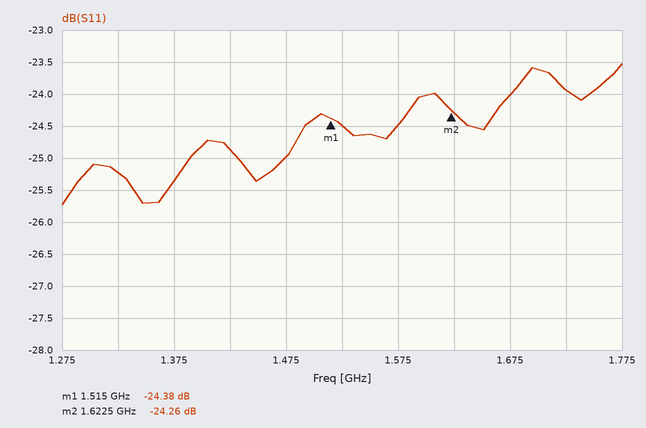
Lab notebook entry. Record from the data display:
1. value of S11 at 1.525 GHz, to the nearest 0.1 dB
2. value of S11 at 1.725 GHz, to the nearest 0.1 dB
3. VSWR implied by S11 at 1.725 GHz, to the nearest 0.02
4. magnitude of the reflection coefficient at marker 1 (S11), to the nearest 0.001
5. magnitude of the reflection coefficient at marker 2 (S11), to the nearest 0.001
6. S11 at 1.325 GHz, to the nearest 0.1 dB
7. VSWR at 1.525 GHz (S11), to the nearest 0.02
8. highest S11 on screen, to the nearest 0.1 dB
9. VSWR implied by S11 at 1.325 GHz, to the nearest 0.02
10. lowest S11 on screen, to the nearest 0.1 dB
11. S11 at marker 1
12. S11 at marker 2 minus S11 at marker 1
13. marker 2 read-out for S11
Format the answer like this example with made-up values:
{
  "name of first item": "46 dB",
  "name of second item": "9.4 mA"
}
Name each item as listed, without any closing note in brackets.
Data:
{
  "value of S11 at 1.525 GHz, to the nearest 0.1 dB": "-24.5 dB",
  "value of S11 at 1.725 GHz, to the nearest 0.1 dB": "-23.9 dB",
  "VSWR implied by S11 at 1.725 GHz, to the nearest 0.02": "1.14",
  "magnitude of the reflection coefficient at marker 1 (S11), to the nearest 0.001": "0.060",
  "magnitude of the reflection coefficient at marker 2 (S11), to the nearest 0.001": "0.061",
  "S11 at 1.325 GHz, to the nearest 0.1 dB": "-25.2 dB",
  "VSWR at 1.525 GHz (S11), to the nearest 0.02": "1.12",
  "highest S11 on screen, to the nearest 0.1 dB": "-23.5 dB",
  "VSWR implied by S11 at 1.325 GHz, to the nearest 0.02": "1.12",
  "lowest S11 on screen, to the nearest 0.1 dB": "-25.7 dB",
  "S11 at marker 1": "-24.38 dB",
  "S11 at marker 2 minus S11 at marker 1": "0.12 dB",
  "marker 2 read-out for S11": "-24.26 dB"
}
